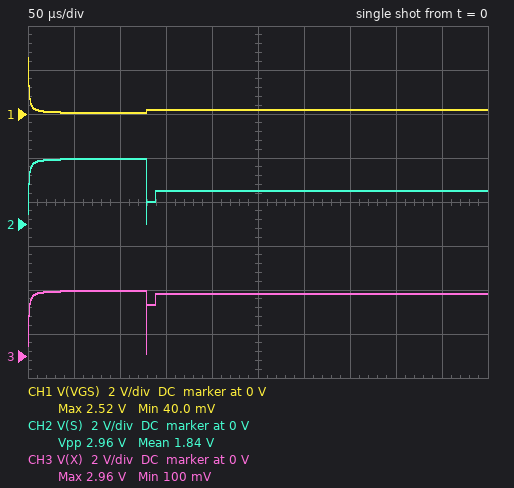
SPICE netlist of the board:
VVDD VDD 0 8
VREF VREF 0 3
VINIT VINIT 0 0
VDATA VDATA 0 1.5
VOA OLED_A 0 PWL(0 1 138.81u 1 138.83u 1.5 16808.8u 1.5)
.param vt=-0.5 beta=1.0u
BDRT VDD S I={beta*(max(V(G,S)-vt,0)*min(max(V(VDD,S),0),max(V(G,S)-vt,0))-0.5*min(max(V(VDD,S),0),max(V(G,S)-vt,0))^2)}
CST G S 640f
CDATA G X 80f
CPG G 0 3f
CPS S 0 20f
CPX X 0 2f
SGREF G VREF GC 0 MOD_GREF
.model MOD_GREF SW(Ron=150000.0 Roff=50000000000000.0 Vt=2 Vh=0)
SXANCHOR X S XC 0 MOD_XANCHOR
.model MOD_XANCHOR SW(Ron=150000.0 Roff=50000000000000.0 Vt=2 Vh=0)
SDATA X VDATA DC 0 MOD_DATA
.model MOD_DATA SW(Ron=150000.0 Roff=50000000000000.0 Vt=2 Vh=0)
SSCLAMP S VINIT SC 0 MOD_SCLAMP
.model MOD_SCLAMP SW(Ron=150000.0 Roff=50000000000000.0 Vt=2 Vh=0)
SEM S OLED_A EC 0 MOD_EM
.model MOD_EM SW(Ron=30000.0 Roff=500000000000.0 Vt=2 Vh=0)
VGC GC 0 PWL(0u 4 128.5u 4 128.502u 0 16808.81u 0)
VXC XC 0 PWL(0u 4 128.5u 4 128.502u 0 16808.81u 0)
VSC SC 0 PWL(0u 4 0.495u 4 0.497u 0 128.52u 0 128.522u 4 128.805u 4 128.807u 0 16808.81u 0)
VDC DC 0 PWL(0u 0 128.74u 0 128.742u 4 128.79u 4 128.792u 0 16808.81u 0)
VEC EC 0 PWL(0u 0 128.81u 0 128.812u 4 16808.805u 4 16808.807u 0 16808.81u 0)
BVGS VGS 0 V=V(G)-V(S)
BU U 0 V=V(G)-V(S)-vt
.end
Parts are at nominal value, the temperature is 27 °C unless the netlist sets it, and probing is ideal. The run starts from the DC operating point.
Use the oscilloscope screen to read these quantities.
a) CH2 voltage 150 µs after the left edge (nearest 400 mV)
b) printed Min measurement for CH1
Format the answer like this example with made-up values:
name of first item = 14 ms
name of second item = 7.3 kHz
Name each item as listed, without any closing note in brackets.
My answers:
CH2 voltage 150 µs after the left edge = 1.6 V
printed Min measurement for CH1 = 40.0 mV
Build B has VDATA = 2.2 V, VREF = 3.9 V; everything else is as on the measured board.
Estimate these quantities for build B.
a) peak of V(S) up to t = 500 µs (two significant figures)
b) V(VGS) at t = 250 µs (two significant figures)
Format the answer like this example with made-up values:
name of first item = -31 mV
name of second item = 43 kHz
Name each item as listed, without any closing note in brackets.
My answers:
peak of V(S) up to t = 500 µs = 3.9 V
V(VGS) at t = 250 µs = 260 mV
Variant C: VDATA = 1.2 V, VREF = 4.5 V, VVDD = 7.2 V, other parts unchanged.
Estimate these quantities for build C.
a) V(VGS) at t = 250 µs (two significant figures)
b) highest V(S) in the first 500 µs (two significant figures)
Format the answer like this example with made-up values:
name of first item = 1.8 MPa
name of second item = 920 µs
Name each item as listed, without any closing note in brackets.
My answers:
V(VGS) at t = 250 µs = 170 mV
highest V(S) in the first 500 µs = 4.5 V
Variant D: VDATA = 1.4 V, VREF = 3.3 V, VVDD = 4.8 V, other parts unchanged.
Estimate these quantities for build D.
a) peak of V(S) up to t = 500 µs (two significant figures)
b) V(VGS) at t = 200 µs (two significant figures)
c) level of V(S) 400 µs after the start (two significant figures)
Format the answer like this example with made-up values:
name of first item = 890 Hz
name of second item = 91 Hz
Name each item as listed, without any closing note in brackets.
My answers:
peak of V(S) up to t = 500 µs = 3.3 V
V(VGS) at t = 200 µs = 180 mV
level of V(S) 400 µs after the start = 1.5 V
